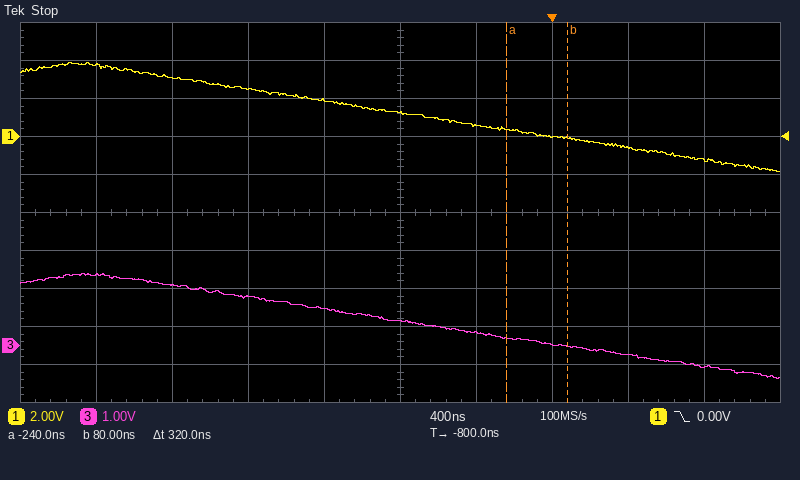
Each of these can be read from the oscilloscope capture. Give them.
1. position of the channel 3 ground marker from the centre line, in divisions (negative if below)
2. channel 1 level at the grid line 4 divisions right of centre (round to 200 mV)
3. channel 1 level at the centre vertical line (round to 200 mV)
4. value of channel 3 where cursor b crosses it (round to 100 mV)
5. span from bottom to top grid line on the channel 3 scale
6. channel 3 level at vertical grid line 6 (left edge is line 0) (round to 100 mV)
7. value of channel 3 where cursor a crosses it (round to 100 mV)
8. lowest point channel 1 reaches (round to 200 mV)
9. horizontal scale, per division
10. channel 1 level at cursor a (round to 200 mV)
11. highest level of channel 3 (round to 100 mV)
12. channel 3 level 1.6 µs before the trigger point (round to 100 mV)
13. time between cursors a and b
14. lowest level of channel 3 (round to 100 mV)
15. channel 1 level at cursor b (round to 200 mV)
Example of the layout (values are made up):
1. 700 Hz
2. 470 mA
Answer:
1. -3.5 div
2. -1.2 V
3. 1.2 V
4. 0.0 V
5. 10 V
6. 300 mV
7. 200 mV
8. -1.8 V
9. 400 ns
10. 400 mV
11. 1.9 V
12. 1.3 V
13. 320 ns
14. -900 mV
15. 0.0 V
